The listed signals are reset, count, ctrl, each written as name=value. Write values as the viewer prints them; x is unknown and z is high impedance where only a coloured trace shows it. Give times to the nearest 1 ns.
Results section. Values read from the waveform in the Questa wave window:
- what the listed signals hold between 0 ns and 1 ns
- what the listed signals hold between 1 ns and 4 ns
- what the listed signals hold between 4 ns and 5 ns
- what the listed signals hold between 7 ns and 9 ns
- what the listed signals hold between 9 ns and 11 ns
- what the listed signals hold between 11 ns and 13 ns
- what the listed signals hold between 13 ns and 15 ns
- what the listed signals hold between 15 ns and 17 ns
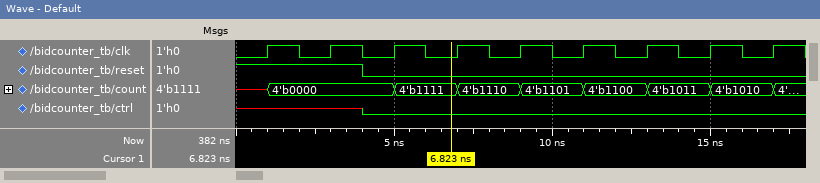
reset=1, count=x, ctrl=x
reset=1, count=4'b0000, ctrl=x
reset=0, count=4'b0000, ctrl=0
reset=0, count=4'b1110, ctrl=0
reset=0, count=4'b1101, ctrl=0
reset=0, count=4'b1100, ctrl=0
reset=0, count=4'b1011, ctrl=0
reset=0, count=4'b1010, ctrl=0
